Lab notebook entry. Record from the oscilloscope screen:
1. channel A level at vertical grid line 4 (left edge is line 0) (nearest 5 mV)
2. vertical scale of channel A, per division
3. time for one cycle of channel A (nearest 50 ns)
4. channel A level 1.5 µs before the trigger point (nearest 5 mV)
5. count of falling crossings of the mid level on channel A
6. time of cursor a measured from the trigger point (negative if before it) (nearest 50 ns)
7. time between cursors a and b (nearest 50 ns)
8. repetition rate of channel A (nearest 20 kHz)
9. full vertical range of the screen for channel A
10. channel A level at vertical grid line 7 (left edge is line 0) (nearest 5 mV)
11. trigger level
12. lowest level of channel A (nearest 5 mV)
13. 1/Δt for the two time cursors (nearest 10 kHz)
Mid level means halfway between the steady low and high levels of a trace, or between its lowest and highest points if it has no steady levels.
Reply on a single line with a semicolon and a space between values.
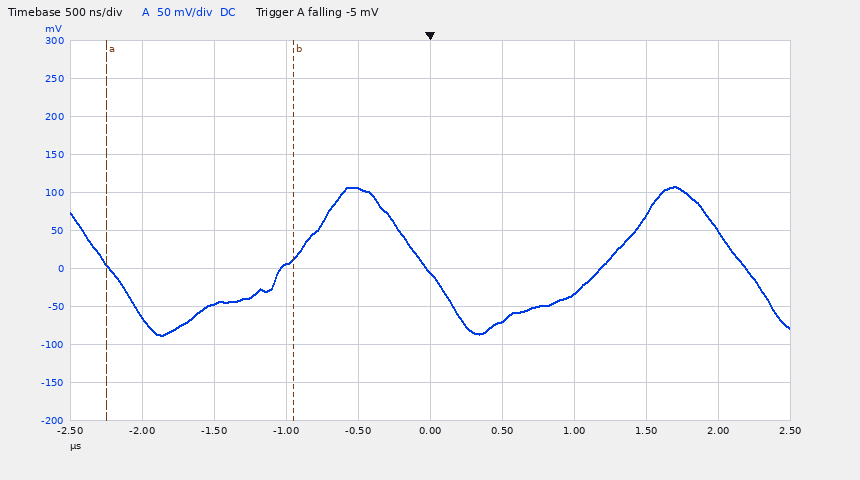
105 mV; 50 mV; 2.20 µs; -45 mV; 3; -2.25 µs; 1.30 µs; 460 kHz; 500 mV; -35 mV; -5 mV; -90 mV; 770 kHz
